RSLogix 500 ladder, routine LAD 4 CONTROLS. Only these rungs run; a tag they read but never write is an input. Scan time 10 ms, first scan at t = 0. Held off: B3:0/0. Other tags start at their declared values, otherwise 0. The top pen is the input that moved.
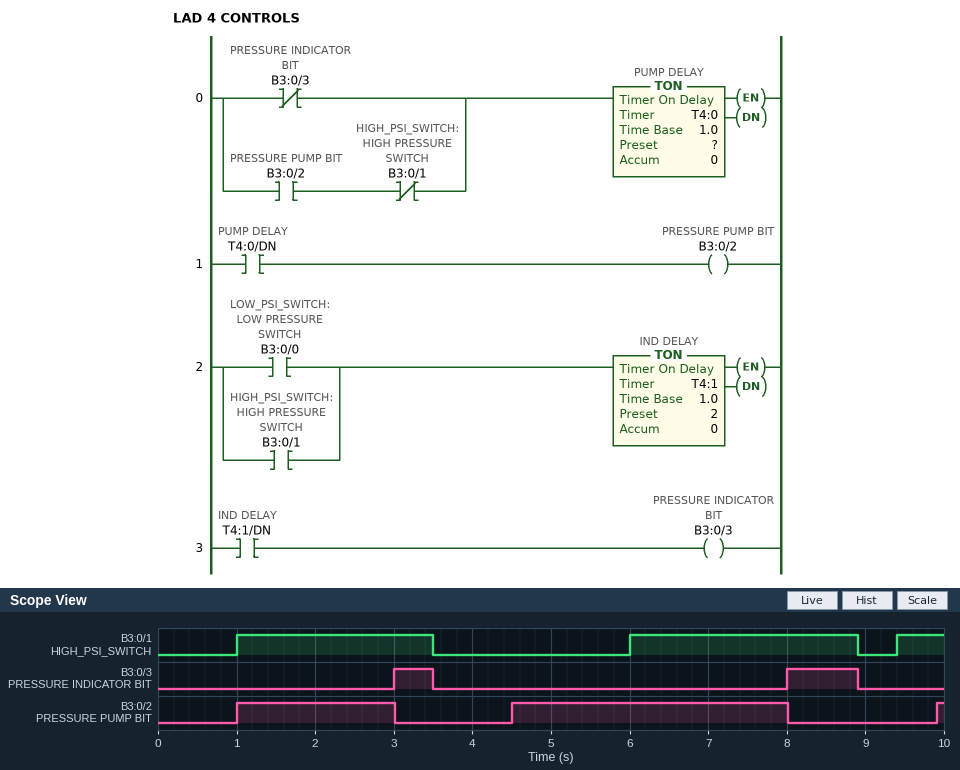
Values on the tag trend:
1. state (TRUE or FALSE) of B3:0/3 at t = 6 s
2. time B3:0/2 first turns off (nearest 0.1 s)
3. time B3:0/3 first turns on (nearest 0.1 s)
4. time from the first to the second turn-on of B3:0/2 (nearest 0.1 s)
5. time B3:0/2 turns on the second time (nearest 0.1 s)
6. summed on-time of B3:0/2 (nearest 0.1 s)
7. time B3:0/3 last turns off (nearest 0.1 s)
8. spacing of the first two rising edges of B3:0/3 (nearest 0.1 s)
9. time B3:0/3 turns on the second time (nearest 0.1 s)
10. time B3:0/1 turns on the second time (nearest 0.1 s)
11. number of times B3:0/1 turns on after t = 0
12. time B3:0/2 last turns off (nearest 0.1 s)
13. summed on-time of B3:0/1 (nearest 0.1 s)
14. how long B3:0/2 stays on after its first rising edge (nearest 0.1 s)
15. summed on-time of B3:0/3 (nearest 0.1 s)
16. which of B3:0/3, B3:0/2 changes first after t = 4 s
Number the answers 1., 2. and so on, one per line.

1. FALSE
2. 3.0 s
3. 3.0 s
4. 3.5 s
5. 4.5 s
6. 5.6 s
7. 8.9 s
8. 5.0 s
9. 8.0 s
10. 6.0 s
11. 3
12. 8.0 s
13. 6.0 s
14. 2.0 s
15. 1.4 s
16. B3:0/2
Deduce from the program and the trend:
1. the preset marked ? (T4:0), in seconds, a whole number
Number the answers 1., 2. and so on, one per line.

1. 1 s
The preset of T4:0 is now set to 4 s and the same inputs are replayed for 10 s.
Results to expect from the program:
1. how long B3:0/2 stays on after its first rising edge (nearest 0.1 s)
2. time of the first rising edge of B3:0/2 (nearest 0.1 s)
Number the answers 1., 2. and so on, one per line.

1. 0.5 s
2. 7.5 s
